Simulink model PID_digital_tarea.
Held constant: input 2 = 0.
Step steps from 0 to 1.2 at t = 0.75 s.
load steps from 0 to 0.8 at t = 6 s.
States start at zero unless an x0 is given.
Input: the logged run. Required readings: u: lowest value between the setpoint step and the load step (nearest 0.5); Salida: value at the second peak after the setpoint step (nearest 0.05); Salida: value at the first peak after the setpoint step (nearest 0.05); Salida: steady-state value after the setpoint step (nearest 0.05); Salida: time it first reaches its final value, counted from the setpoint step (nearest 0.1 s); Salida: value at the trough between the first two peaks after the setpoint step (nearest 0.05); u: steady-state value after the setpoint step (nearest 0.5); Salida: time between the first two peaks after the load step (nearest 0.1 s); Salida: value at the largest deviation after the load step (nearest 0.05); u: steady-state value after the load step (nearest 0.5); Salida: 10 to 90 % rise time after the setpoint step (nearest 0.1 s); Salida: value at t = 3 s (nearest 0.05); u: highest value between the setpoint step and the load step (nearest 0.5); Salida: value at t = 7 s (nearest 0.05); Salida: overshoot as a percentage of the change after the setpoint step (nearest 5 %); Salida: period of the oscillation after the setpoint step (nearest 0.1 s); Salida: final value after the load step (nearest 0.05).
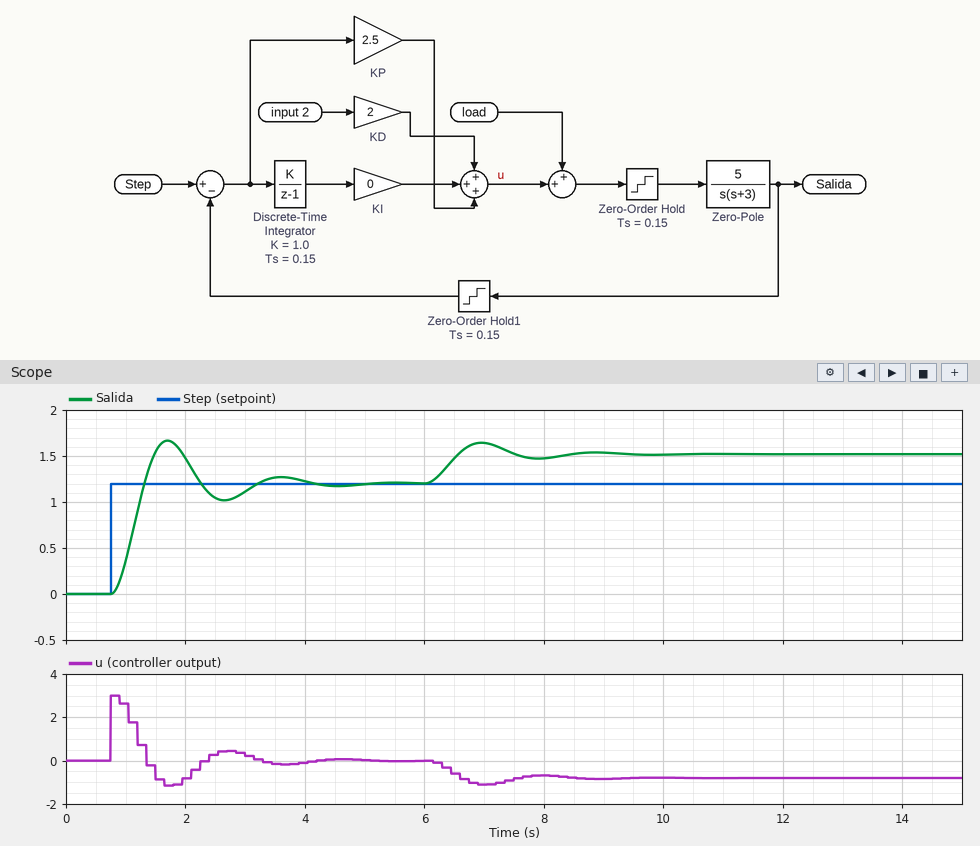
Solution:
-1.0
1.25
1.65
1.20
0.6 s
1.00
0.0
1.9 s
1.65
-1.0
0.4 s
1.10
3.0
1.65
40 %
1.9 s
1.50
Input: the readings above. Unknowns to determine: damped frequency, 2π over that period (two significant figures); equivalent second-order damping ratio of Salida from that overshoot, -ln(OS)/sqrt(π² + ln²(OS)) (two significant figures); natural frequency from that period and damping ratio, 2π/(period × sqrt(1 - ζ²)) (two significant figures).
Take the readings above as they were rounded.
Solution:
3.3 rad/s
0.28
3.4 rad/s
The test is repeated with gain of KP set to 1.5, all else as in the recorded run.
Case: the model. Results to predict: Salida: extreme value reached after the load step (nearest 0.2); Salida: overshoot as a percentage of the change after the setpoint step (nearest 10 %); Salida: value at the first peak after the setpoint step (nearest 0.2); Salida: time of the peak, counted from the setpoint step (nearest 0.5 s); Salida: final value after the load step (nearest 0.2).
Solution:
1.8
20 %
1.4
1.5 s
1.8
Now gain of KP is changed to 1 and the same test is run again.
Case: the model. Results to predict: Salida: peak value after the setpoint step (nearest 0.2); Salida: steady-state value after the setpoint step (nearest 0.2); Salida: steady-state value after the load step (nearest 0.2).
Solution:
1.4
1.2
2.0
